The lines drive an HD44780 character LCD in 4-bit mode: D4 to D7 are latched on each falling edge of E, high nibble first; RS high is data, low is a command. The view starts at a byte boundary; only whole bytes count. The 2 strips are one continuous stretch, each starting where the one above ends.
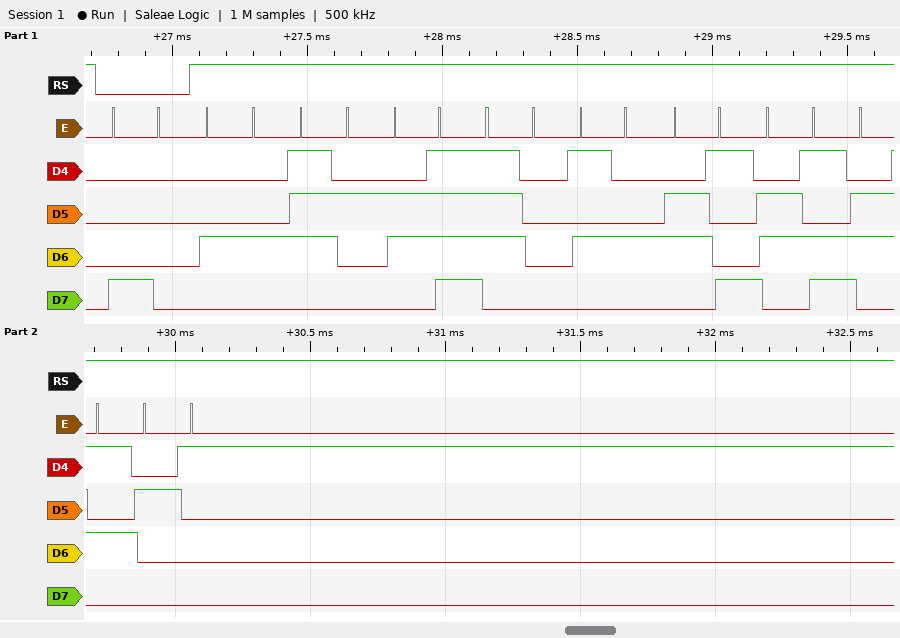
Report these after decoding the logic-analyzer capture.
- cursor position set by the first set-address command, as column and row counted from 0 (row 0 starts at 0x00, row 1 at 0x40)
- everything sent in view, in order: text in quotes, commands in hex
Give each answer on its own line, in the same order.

column 0, row 0
0x80 "DropTime!"
